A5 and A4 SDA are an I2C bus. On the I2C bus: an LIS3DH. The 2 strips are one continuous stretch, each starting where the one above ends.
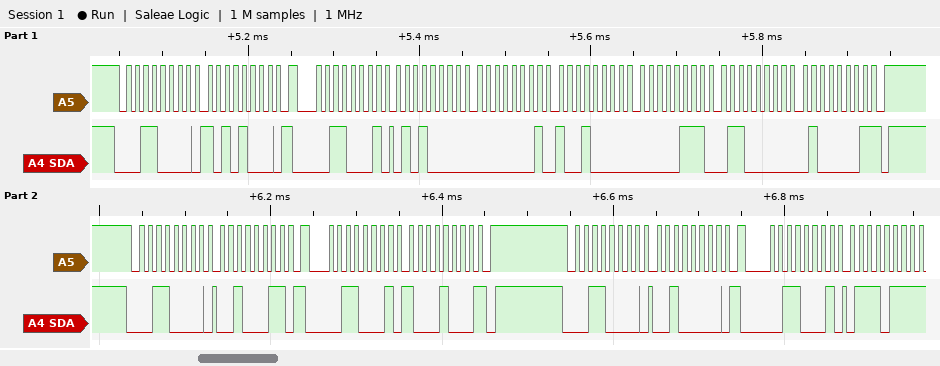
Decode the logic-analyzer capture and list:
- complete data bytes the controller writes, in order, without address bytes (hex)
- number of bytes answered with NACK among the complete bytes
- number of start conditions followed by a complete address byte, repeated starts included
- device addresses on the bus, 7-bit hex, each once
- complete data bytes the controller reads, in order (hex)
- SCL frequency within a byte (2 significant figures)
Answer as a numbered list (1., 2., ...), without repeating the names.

1. A8 23 20
2. 3
3. 6
4. 0x18
5. 50 01 90 07 60 41 88 77
6. 100 kHz
